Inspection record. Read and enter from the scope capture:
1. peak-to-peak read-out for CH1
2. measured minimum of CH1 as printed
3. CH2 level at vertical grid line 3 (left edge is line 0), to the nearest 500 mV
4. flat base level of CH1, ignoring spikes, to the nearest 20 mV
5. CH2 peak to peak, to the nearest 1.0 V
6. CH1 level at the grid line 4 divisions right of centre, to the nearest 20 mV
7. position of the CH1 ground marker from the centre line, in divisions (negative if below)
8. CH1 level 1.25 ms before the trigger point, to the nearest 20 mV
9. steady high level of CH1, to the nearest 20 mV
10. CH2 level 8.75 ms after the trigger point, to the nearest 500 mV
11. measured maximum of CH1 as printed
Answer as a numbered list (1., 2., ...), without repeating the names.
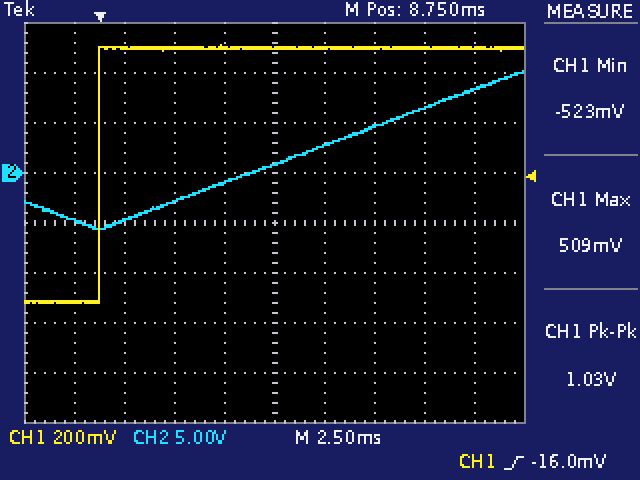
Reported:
1. 1.03 V
2. -523 mV
3. -3.0 V
4. -520 mV
5. 16.0 V
6. 500 mV
7. +1.0 div
8. -520 mV
9. 500 mV
10. 1.0 V
11. 509 mV
